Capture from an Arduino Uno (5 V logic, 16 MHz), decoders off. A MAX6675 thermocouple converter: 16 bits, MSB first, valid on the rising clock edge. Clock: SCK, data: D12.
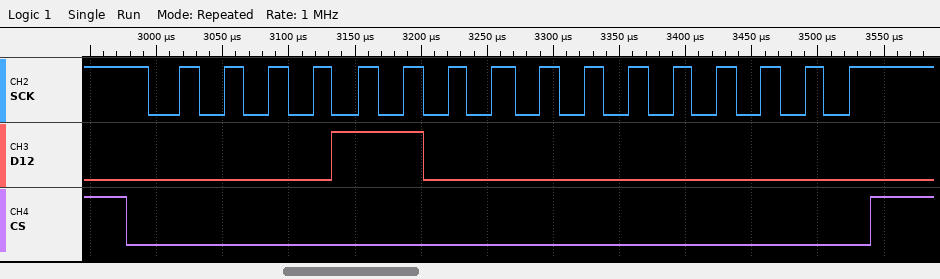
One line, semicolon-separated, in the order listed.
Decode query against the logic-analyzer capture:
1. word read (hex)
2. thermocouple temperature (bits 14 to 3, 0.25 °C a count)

0x0C00; 96.00 °C
